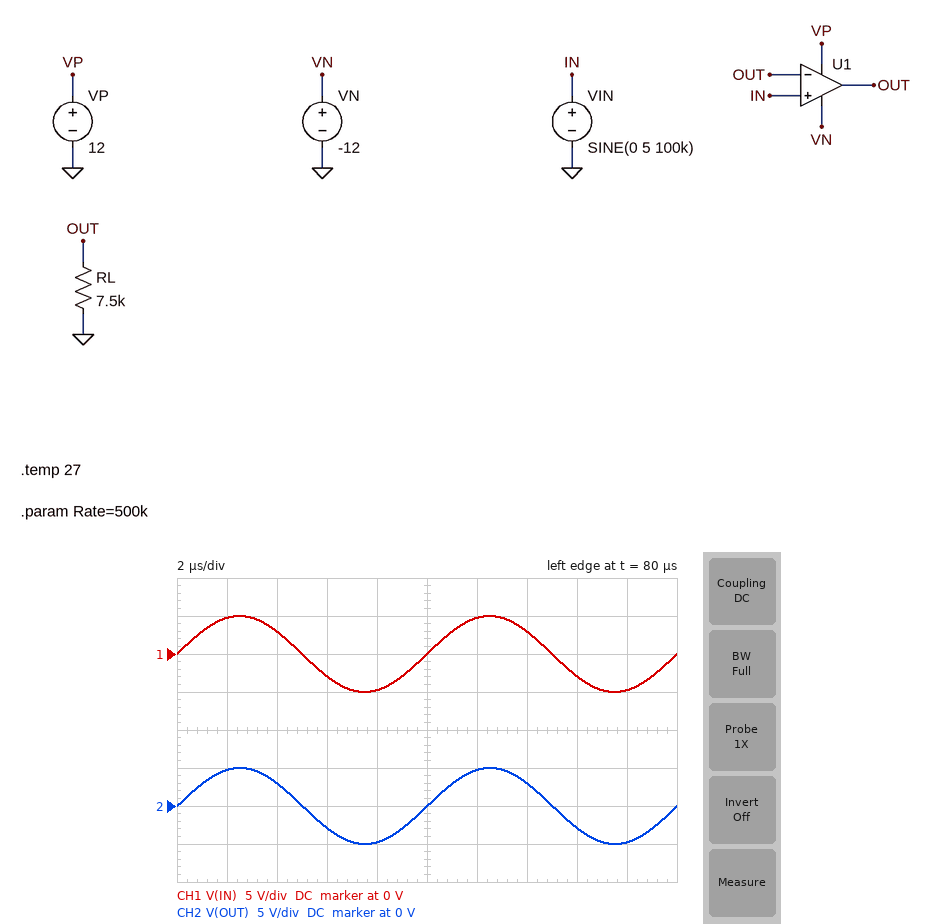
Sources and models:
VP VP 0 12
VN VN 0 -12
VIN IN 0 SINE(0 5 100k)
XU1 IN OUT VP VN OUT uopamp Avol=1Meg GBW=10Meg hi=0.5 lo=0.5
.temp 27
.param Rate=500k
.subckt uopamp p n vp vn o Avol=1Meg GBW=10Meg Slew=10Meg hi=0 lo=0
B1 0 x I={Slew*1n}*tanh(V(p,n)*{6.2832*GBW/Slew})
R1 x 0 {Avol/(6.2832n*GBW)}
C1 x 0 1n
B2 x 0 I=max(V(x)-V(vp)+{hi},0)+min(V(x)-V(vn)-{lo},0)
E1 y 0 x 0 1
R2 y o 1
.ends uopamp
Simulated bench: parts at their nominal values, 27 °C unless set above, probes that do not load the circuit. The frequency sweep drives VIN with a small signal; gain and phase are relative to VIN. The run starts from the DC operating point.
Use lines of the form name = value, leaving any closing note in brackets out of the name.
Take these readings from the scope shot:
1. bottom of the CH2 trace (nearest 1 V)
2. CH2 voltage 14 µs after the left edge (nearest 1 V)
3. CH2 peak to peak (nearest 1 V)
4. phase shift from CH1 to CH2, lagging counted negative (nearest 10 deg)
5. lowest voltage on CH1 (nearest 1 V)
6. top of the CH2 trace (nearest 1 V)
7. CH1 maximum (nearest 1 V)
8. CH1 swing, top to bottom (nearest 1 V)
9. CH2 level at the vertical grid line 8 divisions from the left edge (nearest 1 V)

bottom of the CH2 trace = -5 V
CH2 voltage 14 µs after the left edge = 3 V
CH2 peak to peak = 10 V
phase shift from CH1 to CH2, lagging counted negative = 0 deg
lowest voltage on CH1 = -5 V
top of the CH2 trace = 5 V
CH1 maximum = 5 V
CH1 swing, top to bottom = 10 V
CH2 level at the vertical grid line 8 divisions from the left edge = -3 V
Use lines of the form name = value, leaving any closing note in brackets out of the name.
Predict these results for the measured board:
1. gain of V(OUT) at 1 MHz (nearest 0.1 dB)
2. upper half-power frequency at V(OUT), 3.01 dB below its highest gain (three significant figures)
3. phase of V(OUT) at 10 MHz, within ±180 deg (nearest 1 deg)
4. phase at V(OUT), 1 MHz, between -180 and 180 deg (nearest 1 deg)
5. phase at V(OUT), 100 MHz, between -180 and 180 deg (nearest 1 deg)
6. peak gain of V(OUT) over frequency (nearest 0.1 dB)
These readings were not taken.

gain of V(OUT) at 1 MHz = 0 dB
upper half-power frequency at V(OUT), 3.01 dB below its highest gain = 10.0 MHz
phase of V(OUT) at 10 MHz, within ±180 deg = -45 deg
phase at V(OUT), 1 MHz, between -180 and 180 deg = -6 deg
phase at V(OUT), 100 MHz, between -180 and 180 deg = -84 deg
peak gain of V(OUT) over frequency = 0 dB
